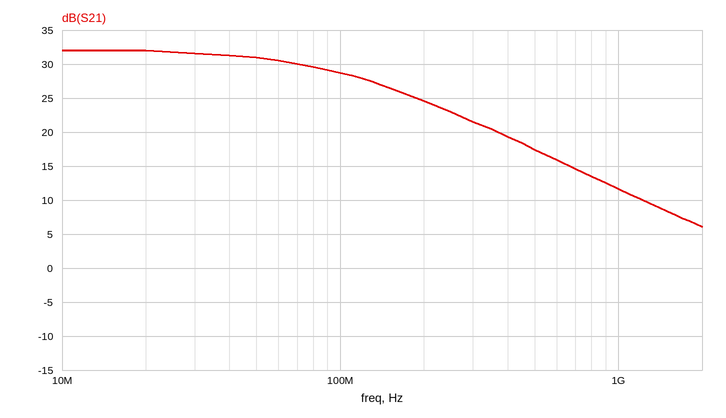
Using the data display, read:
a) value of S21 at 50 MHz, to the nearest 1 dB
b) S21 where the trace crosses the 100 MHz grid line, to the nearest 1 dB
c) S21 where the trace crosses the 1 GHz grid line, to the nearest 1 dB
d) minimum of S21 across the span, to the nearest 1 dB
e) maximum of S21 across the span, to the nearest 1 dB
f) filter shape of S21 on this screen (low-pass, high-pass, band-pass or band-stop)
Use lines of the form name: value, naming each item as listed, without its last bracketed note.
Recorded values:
value of S21 at 50 MHz, to the nearest 1 dB: 31 dB
S21 where the trace crosses the 100 MHz grid line, to the nearest 1 dB: 29 dB
S21 where the trace crosses the 1 GHz grid line, to the nearest 1 dB: 12 dB
minimum of S21 across the span, to the nearest 1 dB: 6 dB
maximum of S21 across the span, to the nearest 1 dB: 32 dB
filter shape of S21 on this screen: low-pass
